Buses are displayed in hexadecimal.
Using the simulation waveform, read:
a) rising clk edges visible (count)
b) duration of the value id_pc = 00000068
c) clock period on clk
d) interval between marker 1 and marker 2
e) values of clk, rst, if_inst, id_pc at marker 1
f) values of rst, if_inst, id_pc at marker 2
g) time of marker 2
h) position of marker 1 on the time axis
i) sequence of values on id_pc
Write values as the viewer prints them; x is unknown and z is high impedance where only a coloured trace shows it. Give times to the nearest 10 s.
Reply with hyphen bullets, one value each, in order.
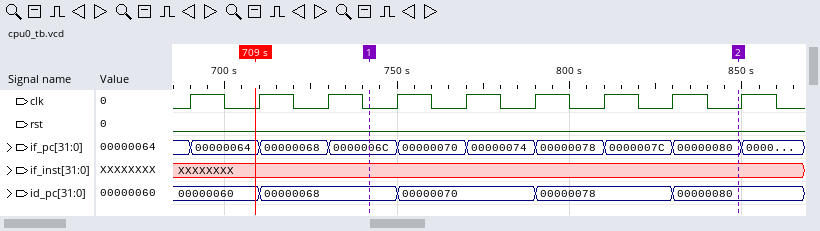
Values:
- 9
- 40 s
- 20 s
- 110 s
- clk=0, rst=0, if_inst=XXXXXXXX, id_pc=00000068
- rst=0, if_inst=XXXXXXXX, id_pc=00000080
- 850 s
- 740 s
- 00000060, 00000068, 00000070, 00000078, 00000080
